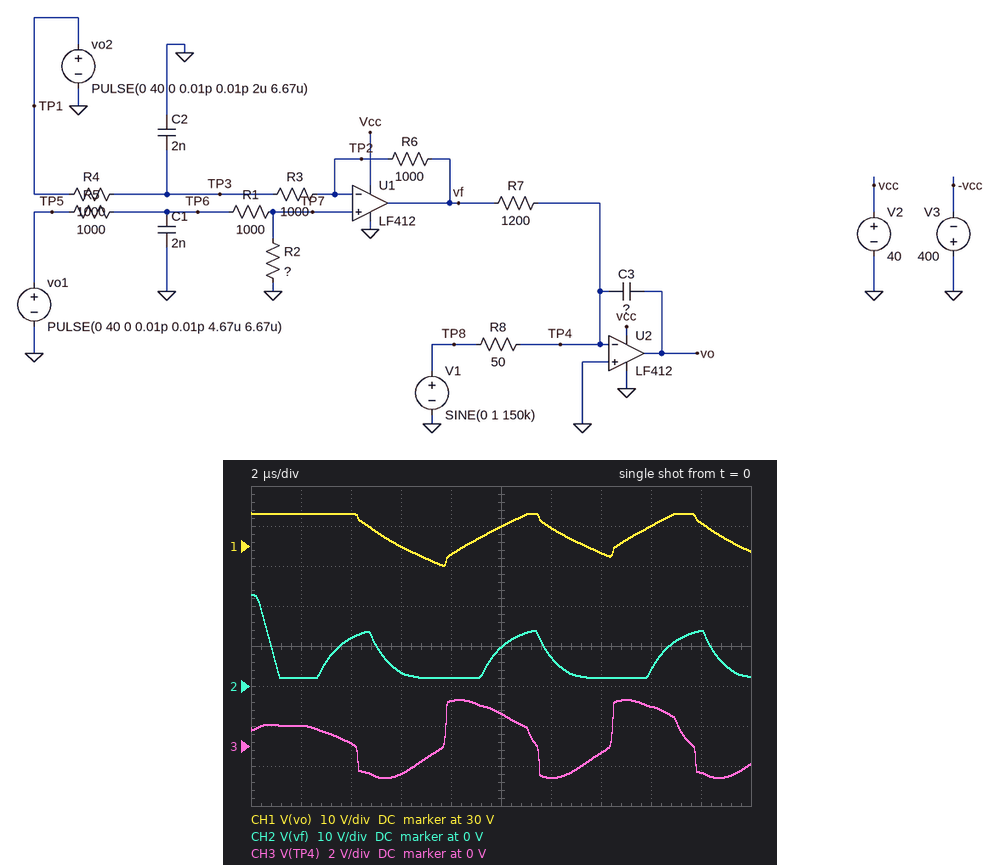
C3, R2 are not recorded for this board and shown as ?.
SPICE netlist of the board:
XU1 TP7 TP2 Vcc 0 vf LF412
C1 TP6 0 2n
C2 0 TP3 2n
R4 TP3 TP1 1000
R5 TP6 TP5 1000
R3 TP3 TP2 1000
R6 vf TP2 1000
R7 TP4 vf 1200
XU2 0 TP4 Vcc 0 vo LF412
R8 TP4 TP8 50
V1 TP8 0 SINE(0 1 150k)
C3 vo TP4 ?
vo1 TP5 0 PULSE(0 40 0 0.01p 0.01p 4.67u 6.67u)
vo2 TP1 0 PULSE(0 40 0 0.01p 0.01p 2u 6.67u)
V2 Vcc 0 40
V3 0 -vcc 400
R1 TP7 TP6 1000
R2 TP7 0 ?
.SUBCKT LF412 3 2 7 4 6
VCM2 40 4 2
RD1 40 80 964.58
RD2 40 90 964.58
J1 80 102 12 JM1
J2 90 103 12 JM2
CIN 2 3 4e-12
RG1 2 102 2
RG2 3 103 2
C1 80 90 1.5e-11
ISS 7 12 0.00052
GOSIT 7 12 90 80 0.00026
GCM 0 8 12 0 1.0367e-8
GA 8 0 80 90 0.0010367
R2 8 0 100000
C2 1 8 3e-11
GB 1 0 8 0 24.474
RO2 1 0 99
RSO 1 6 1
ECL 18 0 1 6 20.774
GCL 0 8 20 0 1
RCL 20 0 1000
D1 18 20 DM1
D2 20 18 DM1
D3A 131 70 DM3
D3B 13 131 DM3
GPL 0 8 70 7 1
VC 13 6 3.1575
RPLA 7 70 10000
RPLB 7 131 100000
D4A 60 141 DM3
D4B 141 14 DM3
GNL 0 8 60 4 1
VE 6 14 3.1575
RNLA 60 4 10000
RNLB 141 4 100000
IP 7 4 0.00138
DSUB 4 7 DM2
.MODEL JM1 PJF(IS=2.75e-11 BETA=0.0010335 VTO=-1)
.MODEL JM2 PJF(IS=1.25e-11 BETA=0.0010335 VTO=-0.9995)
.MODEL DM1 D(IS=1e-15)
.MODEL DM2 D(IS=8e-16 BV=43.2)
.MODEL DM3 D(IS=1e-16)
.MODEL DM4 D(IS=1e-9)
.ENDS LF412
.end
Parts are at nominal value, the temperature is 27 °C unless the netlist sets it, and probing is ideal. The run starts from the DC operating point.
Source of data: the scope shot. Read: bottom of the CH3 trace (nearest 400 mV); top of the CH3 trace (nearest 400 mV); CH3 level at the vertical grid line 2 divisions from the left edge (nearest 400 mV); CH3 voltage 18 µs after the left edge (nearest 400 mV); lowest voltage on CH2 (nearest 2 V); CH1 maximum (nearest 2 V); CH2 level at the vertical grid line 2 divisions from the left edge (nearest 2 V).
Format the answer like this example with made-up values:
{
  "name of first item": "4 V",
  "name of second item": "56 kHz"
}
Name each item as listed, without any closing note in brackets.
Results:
{
  "bottom of the CH3 trace": "-1.6 V",
  "top of the CH3 trace": "2.4 V",
  "CH3 level at the vertical grid line 2 divisions from the left edge": "0 V",
  "CH3 voltage 18 µs after the left edge": "-1.2 V",
  "lowest voltage on CH2": "2 V",
  "CH1 maximum": "38 V",
  "CH2 level at the vertical grid line 2 divisions from the left edge": "12 V"
}
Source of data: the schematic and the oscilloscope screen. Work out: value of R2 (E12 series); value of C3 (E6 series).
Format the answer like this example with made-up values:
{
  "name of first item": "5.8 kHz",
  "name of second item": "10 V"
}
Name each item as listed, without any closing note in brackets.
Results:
{
  "value of R2": "680 Ω",
  "value of C3": "6.8 nF"
}
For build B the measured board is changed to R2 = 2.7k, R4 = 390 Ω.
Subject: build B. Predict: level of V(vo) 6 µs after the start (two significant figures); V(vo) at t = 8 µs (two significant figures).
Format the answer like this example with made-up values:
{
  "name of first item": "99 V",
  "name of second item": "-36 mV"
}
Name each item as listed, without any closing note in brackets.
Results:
{
  "level of V(vo) 6 µs after the start": "33 V",
  "V(vo) at t = 8 µs": "30 V"
}
